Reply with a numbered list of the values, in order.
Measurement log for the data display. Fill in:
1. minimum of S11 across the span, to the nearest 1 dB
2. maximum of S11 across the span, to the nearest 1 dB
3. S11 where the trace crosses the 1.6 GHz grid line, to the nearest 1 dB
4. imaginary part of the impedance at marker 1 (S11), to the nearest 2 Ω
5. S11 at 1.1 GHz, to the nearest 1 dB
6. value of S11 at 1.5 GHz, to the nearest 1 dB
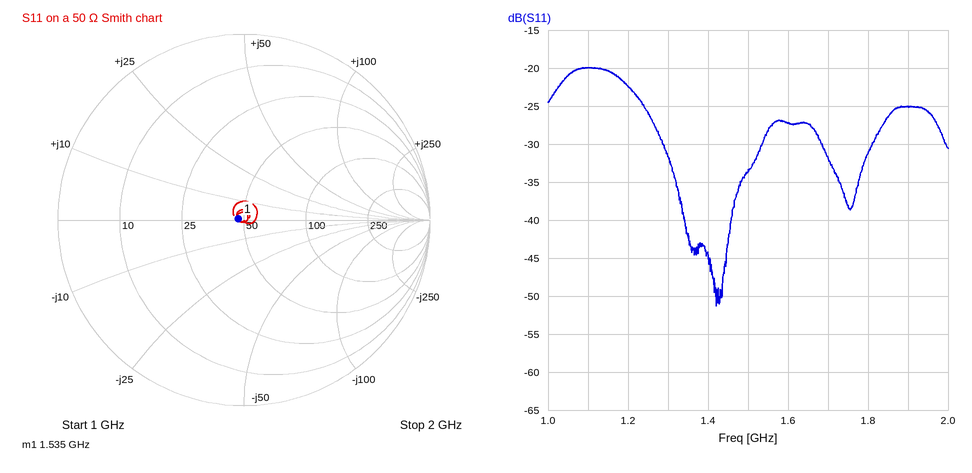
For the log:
1. -51 dB
2. -20 dB
3. -27 dB
4. 0 Ω
5. -20 dB
6. -34 dB
